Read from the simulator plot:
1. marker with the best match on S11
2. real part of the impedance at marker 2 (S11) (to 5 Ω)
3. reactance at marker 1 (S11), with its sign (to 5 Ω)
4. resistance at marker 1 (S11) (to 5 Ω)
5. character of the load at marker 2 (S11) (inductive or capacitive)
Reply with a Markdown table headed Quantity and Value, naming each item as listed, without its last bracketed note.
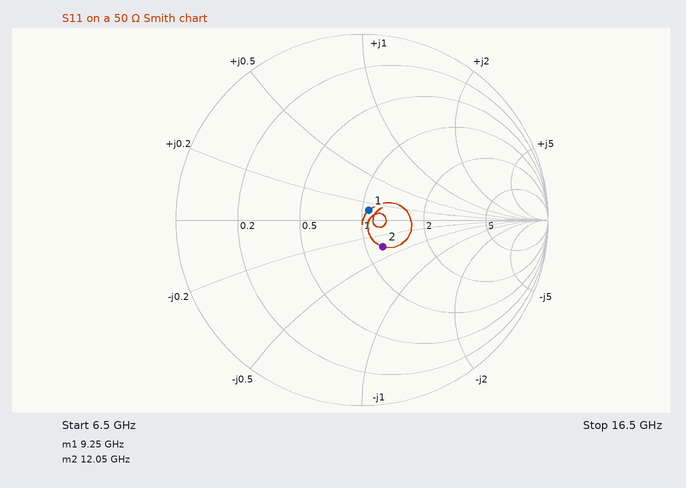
| Quantity | Value |
|---|---|
| marker with the best match on S11 | marker 1 |
| real part of the impedance at marker 2 (S11) | 60 Ω |
| reactance at marker 1 (S11), with its sign | +5 Ω |
| resistance at marker 1 (S11) | 55 Ω |
| character of the load at marker 2 (S11) | capacitive |
